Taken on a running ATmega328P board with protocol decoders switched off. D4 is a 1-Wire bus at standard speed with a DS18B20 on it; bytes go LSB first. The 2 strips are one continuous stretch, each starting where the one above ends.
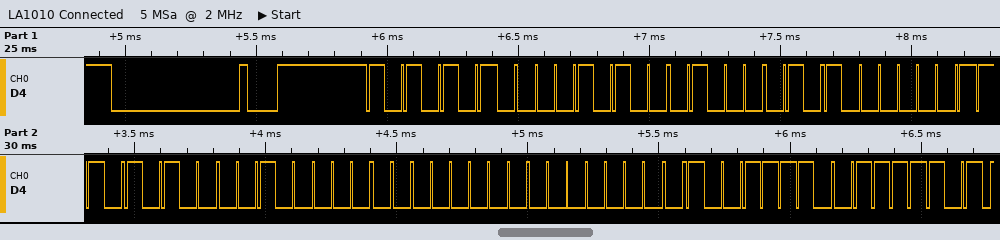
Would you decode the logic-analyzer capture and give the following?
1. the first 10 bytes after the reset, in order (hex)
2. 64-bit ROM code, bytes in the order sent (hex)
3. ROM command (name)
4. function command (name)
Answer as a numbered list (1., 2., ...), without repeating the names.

1. 55 28 42 81 2B 04 00 00 79 BE
2. 28 42 81 2B 04 00 00 79
3. Match ROM
4. Read Scratchpad
